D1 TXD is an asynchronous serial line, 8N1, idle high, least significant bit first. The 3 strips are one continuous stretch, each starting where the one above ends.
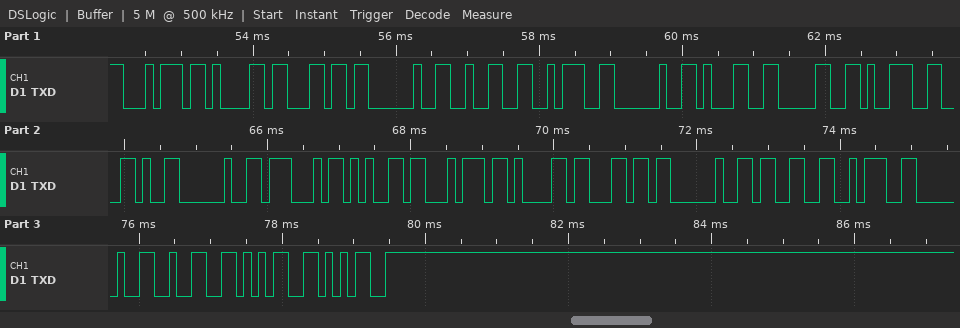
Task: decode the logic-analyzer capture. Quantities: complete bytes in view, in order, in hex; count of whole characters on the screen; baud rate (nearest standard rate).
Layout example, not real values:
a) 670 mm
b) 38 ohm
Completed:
a) 0x74 0x61 0x6C 0x20 0x32 0x3A 0x20 0x31 0x30 0x39 0x2C 0x20 0x47 0x65 0x74 0x61 0x6C 0x20 0x33 0x3A 0x20 0x32 0x35 0x35
b) 24
c) 9600 baud
